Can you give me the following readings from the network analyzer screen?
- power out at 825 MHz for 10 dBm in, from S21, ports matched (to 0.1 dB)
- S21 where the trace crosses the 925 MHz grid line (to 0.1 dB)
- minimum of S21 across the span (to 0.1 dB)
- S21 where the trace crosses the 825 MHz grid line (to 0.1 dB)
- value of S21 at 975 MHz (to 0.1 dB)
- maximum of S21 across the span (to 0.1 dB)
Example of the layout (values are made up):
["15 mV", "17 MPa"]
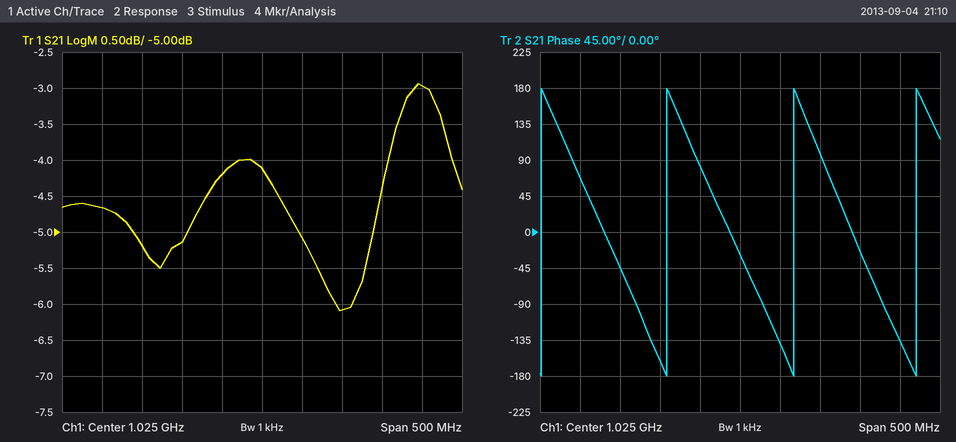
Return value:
["5.3 dBm", "-5.1 dB", "-6.1 dB", "-4.7 dB", "-4.2 dB", "-2.9 dB"]
